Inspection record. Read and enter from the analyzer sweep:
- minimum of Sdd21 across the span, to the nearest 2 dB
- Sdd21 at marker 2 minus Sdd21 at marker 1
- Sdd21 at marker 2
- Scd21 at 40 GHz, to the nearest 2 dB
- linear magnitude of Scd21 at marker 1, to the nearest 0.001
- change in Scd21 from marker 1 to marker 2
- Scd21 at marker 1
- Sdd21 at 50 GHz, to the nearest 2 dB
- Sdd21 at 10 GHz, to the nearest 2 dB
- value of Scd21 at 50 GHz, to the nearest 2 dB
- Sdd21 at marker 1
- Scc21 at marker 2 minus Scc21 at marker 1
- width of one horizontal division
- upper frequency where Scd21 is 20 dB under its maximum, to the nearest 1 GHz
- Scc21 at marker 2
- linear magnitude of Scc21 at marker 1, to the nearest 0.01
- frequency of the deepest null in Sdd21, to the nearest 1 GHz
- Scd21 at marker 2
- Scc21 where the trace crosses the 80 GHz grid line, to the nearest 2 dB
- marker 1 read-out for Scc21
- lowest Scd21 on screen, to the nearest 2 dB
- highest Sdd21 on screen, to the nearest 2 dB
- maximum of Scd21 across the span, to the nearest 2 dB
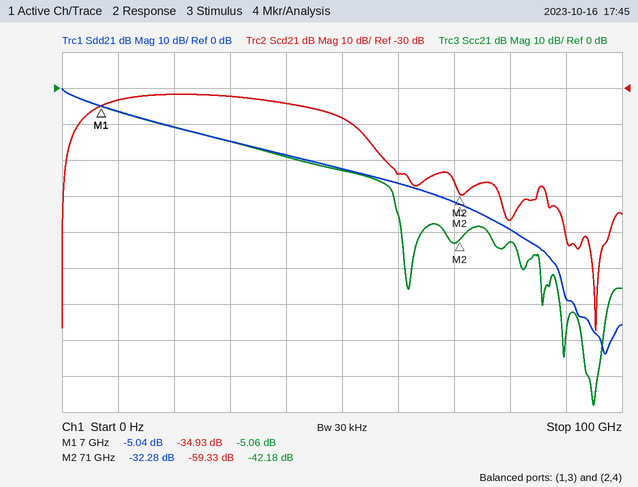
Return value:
-74 dB
-27.24 dB
-32.28 dB
-34 dB
0.018
-24.40 dB
-34.93 dB
-22 dB
-6 dB
-38 dB
-5.04 dB
-37.12 dB
10 GHz
59 GHz
-42.18 dB
0.56
97 GHz
-59.33 dB
-42 dB
-5.06 dB
-98 dB
0 dB
-32 dB
